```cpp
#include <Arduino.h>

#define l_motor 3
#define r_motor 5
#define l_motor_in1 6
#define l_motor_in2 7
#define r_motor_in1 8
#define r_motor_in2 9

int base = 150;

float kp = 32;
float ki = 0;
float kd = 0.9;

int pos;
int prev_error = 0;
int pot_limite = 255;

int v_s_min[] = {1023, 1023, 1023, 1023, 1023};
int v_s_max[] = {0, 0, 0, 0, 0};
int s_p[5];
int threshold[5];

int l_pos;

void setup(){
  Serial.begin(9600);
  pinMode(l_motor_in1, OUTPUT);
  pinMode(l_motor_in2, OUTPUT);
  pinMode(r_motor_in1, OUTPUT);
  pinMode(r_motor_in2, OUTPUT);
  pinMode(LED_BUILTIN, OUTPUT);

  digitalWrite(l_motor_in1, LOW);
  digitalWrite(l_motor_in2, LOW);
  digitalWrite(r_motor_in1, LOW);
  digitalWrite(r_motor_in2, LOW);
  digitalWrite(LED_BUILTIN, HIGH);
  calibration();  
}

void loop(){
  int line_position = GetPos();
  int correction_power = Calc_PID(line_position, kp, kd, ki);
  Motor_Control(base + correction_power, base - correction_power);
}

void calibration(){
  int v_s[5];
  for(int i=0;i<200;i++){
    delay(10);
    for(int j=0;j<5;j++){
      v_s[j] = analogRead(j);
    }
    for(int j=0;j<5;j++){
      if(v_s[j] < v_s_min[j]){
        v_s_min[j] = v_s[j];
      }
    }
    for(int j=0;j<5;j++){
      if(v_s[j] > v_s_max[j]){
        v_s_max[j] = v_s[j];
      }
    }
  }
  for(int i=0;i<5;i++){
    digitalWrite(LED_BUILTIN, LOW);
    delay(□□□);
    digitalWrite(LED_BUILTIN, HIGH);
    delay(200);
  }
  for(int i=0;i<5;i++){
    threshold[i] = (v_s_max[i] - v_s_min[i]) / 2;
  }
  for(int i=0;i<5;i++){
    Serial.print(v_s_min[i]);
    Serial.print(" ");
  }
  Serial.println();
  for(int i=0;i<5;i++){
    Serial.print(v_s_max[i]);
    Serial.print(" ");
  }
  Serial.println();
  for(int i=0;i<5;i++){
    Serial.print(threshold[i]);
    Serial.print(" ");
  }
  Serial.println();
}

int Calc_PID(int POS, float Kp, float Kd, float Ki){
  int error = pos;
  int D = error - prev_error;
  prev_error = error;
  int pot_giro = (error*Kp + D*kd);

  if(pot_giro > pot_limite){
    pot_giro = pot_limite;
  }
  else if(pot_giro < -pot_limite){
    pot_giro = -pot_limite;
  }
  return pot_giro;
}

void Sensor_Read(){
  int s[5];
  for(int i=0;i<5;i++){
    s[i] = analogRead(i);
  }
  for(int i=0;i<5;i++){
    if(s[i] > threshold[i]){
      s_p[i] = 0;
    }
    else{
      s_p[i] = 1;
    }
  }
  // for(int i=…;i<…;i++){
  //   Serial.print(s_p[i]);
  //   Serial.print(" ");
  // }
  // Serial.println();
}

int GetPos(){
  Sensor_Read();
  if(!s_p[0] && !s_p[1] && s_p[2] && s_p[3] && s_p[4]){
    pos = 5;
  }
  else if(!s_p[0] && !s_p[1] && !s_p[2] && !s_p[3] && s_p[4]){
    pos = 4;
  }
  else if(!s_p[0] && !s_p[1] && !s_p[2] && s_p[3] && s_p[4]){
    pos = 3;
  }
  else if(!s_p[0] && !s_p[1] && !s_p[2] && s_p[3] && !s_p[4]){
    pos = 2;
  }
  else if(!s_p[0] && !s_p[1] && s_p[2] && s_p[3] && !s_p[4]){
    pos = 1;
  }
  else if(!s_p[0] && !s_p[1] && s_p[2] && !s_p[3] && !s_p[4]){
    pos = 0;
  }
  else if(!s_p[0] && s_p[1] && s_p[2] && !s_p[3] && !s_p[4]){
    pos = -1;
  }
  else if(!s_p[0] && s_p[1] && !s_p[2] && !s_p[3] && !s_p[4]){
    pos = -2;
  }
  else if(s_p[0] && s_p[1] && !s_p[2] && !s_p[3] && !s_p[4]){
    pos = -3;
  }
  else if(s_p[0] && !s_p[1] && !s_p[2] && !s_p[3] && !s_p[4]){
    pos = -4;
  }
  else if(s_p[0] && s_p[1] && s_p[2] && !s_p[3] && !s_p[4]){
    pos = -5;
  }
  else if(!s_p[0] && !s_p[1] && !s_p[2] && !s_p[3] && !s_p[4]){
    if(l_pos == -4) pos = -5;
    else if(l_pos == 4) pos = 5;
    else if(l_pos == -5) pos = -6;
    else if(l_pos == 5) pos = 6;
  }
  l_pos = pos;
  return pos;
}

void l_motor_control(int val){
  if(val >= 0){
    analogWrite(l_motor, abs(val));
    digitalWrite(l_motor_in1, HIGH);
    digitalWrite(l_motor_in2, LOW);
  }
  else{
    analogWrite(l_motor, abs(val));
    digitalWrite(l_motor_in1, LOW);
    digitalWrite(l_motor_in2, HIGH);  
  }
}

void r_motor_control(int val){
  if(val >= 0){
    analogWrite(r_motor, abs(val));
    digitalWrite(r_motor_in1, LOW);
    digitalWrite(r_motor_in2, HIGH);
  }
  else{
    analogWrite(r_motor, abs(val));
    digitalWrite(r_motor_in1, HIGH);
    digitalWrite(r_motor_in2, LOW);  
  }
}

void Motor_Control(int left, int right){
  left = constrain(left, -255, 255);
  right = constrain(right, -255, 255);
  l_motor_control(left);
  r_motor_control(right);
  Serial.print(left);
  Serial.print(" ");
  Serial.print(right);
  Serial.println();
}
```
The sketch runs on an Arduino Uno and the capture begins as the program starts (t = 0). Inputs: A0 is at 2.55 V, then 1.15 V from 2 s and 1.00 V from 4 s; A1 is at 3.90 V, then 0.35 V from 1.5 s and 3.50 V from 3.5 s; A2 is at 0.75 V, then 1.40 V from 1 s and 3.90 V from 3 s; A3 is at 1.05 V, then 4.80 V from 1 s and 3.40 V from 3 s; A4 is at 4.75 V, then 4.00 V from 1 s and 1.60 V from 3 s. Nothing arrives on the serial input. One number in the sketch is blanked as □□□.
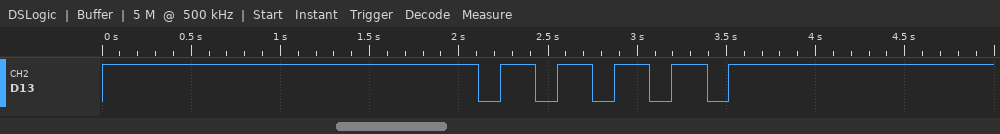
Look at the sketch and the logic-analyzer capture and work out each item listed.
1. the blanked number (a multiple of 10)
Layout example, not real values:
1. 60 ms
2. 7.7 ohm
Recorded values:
1. 120
